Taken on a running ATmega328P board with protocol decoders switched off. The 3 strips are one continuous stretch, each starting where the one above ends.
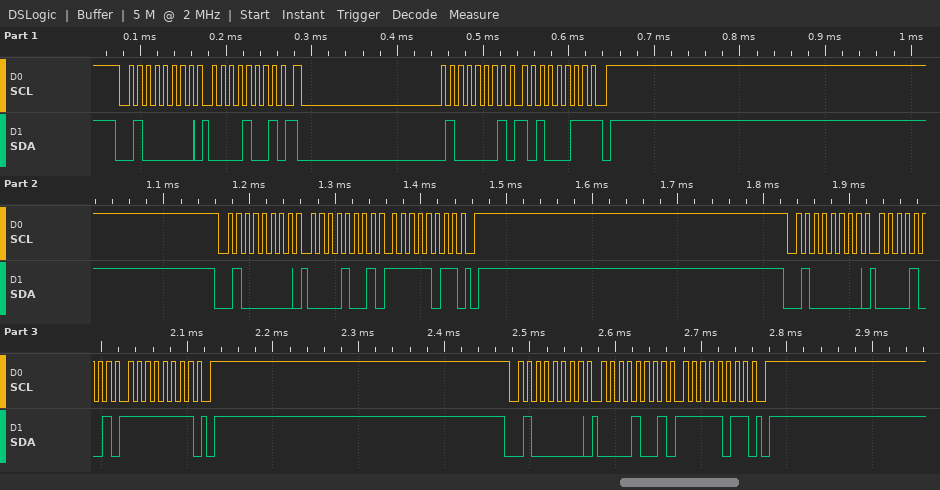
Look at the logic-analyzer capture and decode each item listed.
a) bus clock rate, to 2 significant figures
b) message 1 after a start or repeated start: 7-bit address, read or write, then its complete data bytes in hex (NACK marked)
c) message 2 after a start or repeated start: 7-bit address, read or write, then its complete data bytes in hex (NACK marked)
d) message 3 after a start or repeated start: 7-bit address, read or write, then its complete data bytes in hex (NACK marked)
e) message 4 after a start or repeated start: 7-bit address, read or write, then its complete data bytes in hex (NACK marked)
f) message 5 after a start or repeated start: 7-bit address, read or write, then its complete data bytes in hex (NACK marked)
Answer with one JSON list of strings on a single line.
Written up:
["100 kHz", "0x20 write: 09", "0x20 read: A3 NACK", "0x20 write: 09 FB", "0x20 write: 09 FF", "0x20 write: 09 FB"]
